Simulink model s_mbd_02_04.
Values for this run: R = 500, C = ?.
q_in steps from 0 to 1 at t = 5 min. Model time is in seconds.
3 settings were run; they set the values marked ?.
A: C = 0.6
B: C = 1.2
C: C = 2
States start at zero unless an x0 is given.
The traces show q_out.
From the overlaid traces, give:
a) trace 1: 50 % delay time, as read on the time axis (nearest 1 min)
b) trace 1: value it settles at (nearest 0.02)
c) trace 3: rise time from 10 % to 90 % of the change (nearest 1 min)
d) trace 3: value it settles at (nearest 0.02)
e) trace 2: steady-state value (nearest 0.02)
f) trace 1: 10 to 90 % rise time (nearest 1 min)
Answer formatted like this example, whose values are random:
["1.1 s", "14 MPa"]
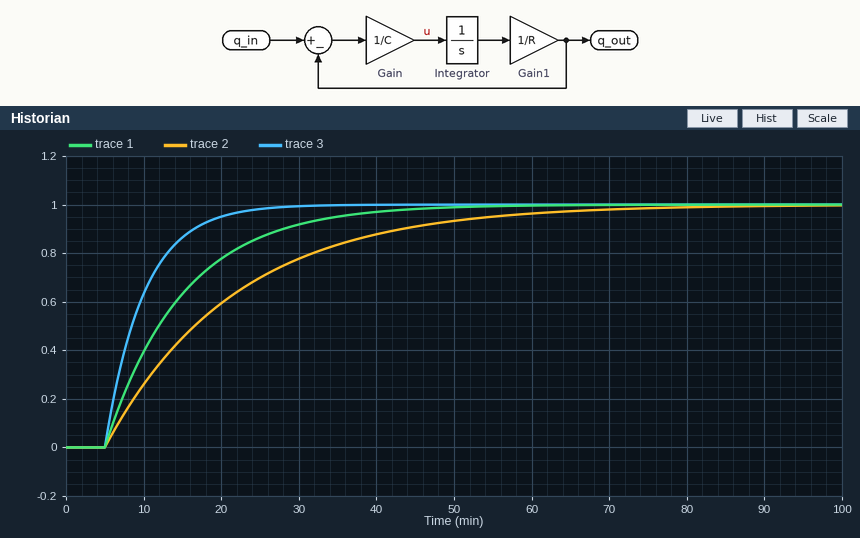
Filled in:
["12 min", "1.00", "11 min", "1.00", "1.00", "22 min"]
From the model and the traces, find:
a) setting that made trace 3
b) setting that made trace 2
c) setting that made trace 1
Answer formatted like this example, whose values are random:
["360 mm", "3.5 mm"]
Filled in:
["A", "C", "B"]
